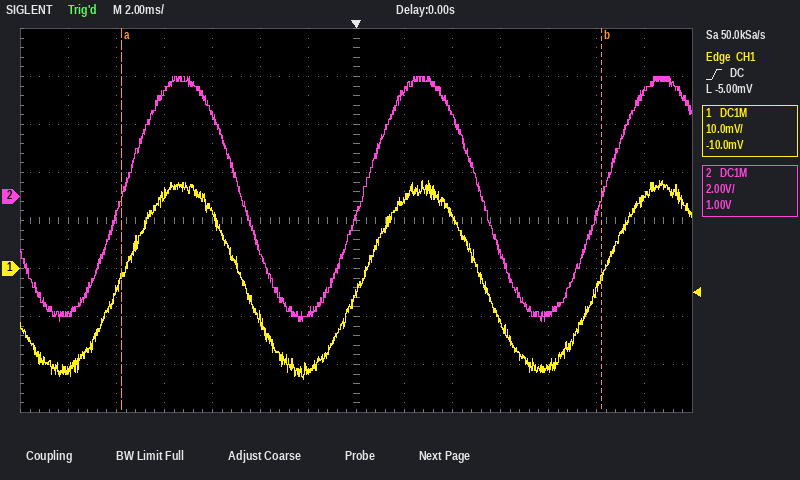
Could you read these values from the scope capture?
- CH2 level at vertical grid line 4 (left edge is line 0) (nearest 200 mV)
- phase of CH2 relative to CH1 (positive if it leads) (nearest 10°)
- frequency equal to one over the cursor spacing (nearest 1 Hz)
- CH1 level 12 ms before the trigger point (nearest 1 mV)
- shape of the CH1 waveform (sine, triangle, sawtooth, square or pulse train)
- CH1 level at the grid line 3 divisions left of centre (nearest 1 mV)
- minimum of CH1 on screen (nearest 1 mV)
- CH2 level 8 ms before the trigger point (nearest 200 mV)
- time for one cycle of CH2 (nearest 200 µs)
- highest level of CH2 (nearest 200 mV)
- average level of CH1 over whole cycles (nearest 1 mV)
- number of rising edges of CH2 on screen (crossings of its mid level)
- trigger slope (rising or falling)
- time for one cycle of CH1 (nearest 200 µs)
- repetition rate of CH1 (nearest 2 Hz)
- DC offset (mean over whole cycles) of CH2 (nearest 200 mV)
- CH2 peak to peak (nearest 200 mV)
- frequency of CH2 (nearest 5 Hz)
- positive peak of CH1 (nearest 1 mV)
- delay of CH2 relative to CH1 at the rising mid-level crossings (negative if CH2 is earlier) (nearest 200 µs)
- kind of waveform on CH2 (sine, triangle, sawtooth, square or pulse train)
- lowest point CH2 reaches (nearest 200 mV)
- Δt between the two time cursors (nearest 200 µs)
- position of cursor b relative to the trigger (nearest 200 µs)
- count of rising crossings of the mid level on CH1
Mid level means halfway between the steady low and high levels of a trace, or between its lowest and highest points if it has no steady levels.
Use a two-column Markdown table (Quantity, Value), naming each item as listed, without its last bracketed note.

| Quantity | Value |
|---|---|
| CH2 level at vertical grid line 4 (left edge is line 0) | 3.4 V |
| phase of CH2 relative to CH1 (positive if it leads) | 0° |
| frequency equal to one over the cursor spacing | 50 Hz |
| CH1 level 12 ms before the trigger point | -21 mV |
| shape of the CH1 waveform | sine |
| CH1 level at the grid line 3 divisions left of centre | 12 mV |
| minimum of CH1 on screen | -23 mV |
| CH2 level 8 ms before the trigger point | 4.4 V |
| time for one cycle of CH2 | 10.0 ms |
| highest level of CH2 | 5.0 V |
| average level of CH1 over whole cycles | -2 mV |
| number of rising edges of CH2 on screen | 3 |
| trigger slope | rising |
| time for one cycle of CH1 | 10.0 ms |
| repetition rate of CH1 | 100 Hz |
| DC offset (mean over whole cycles) of CH2 | 0.0 V |
| CH2 peak to peak | 10.2 V |
| frequency of CH2 | 100 Hz |
| positive peak of CH1 | 18 mV |
| delay of CH2 relative to CH1 at the rising mid-level crossings (negative if CH2 is earlier) | 0.0 ms |
| kind of waveform on CH2 | sine |
| lowest point CH2 reaches | -5.2 V |
| Δt between the two time cursors | 20.0 ms |
| position of cursor b relative to the trigger | +10.2 ms |
| count of rising crossings of the mid level on CH1 | 3 |
